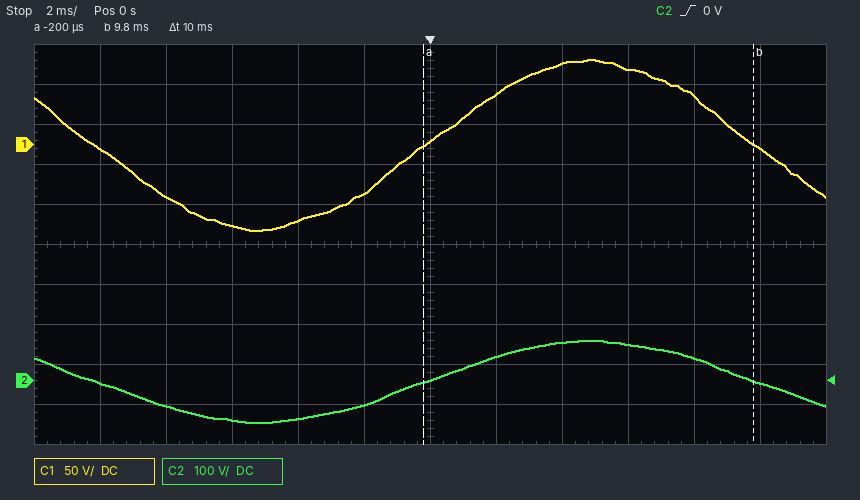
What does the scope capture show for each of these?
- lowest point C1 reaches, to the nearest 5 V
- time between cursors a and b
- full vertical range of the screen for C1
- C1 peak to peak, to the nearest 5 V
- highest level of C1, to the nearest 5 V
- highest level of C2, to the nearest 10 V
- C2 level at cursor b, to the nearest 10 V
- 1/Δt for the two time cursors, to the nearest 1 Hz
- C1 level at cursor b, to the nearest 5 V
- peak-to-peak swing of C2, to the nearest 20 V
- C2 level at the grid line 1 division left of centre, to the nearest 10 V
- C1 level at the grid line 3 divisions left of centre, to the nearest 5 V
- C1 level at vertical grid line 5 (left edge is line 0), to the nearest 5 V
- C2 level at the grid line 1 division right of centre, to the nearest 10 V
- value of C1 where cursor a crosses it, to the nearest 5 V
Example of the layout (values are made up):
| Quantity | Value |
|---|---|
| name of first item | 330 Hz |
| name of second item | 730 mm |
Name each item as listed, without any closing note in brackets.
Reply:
| Quantity | Value |
|---|---|
| lowest point C1 reaches, to the nearest 5 V | -110 V |
| time between cursors a and b | 10 ms |
| full vertical range of the screen for C1 | 500 V |
| C1 peak to peak, to the nearest 5 V | 215 V |
| highest level of C1, to the nearest 5 V | 105 V |
| highest level of C2, to the nearest 10 V | 100 V |
| C2 level at cursor b, to the nearest 10 V | 0 V |
| 1/Δt for the two time cursors, to the nearest 1 Hz | 100 Hz |
| C1 level at cursor b, to the nearest 5 V | 0 V |
| peak-to-peak swing of C2, to the nearest 20 V | 200 V |
| C2 level at the grid line 1 division left of centre, to the nearest 10 V | -60 V |
| C1 level at the grid line 3 divisions left of centre, to the nearest 5 V | -100 V |
| C1 level at vertical grid line 5 (left edge is line 0), to the nearest 5 V | -60 V |
| C2 level at the grid line 1 division right of centre, to the nearest 10 V | 60 V |
| value of C1 where cursor a crosses it, to the nearest 5 V | 0 V |
